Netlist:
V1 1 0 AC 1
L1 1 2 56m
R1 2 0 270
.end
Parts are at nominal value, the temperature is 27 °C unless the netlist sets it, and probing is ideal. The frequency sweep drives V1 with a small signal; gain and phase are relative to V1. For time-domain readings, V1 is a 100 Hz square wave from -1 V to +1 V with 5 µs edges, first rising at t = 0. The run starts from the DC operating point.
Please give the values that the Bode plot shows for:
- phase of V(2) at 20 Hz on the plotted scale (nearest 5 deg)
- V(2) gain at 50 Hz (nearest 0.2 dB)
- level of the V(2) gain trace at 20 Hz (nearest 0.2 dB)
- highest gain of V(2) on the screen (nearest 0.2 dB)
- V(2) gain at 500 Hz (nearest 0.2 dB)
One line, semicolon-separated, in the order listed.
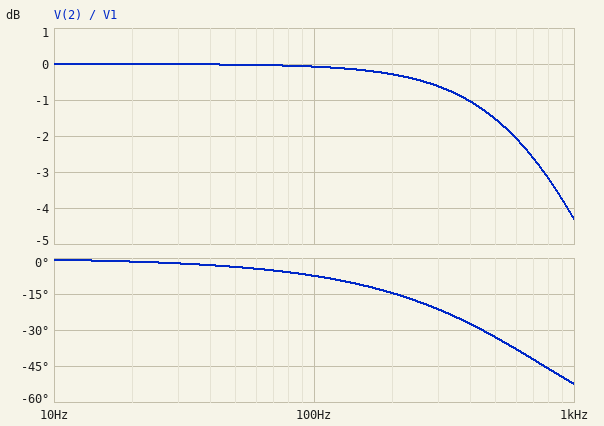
0 deg; 0 dB; 0 dB; 0 dB; -1.6 dB
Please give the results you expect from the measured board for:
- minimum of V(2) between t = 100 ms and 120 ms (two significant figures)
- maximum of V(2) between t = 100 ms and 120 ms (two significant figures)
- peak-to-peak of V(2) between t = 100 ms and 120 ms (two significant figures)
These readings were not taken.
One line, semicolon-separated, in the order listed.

-1.0 V; 1.0 V; 2.0 V
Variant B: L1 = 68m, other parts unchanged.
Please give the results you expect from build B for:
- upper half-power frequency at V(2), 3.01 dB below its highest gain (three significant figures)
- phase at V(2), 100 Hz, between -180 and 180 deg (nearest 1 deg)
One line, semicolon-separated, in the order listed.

632 Hz; -9 deg
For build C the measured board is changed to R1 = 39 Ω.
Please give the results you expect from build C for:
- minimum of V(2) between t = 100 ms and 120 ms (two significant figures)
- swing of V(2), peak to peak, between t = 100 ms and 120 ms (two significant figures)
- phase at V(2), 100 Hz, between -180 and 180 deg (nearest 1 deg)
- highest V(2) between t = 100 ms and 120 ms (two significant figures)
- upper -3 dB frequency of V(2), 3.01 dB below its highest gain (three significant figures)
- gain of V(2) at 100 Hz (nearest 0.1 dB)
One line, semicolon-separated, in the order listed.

-940 mV; 1.9 V; -42 deg; 940 mV; 111 Hz; -2.6 dB
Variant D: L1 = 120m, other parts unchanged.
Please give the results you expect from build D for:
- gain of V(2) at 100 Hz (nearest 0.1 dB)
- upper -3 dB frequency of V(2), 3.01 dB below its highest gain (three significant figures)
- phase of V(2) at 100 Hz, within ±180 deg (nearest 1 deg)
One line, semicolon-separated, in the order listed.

-0.3 dB; 358 Hz; -16 deg
